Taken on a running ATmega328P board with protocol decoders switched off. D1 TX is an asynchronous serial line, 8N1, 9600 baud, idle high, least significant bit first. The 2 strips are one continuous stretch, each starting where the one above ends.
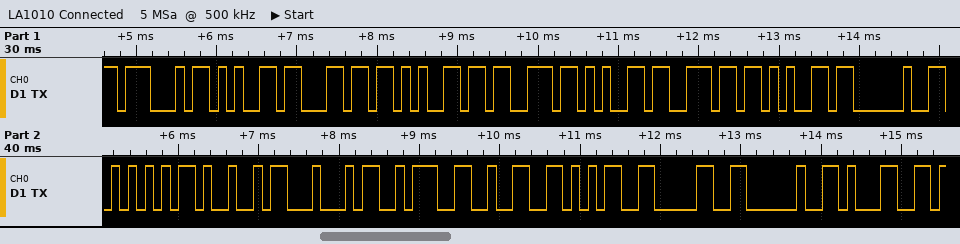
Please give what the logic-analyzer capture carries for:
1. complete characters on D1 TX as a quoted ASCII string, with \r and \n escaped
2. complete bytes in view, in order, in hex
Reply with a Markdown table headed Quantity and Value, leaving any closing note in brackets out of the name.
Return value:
| Quantity | Value |
|---|---|
| complete characters on D1 TX as a quoted ASCII string, with \r and \n escaped | "Gelesene UID:250 1" |
| complete bytes in view, in order, in hex | 0x47 0x65 0x6C 0x65 0x73 0x65 0x6E 0x65 0x20 0x55 0x49 0x44 0x3A 0x32 0x35 0x30 0x20 0x31 |
